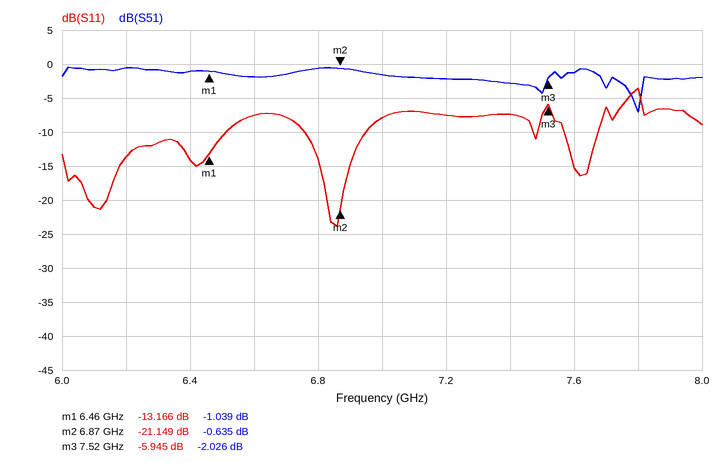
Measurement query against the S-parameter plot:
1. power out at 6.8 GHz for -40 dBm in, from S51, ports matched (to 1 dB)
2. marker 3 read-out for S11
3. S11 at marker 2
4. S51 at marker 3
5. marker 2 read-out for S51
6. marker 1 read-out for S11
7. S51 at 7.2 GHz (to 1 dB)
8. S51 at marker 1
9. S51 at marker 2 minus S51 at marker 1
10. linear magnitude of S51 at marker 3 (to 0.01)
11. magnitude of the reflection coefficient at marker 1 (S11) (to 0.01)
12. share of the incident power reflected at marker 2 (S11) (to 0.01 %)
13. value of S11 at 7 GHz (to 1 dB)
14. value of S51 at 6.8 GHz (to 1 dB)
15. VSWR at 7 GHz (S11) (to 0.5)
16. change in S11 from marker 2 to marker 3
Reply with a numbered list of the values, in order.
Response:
1. -41 dBm
2. -5.945 dB
3. -21.149 dB
4. -2.026 dB
5. -0.635 dB
6. -13.166 dB
7. -2 dB
8. -1.039 dB
9. 0.404 dB
10. 0.79
11. 0.22
12. 0.77 %
13. -8 dB
14. -1 dB
15. 2.5
16. 15.204 dB
